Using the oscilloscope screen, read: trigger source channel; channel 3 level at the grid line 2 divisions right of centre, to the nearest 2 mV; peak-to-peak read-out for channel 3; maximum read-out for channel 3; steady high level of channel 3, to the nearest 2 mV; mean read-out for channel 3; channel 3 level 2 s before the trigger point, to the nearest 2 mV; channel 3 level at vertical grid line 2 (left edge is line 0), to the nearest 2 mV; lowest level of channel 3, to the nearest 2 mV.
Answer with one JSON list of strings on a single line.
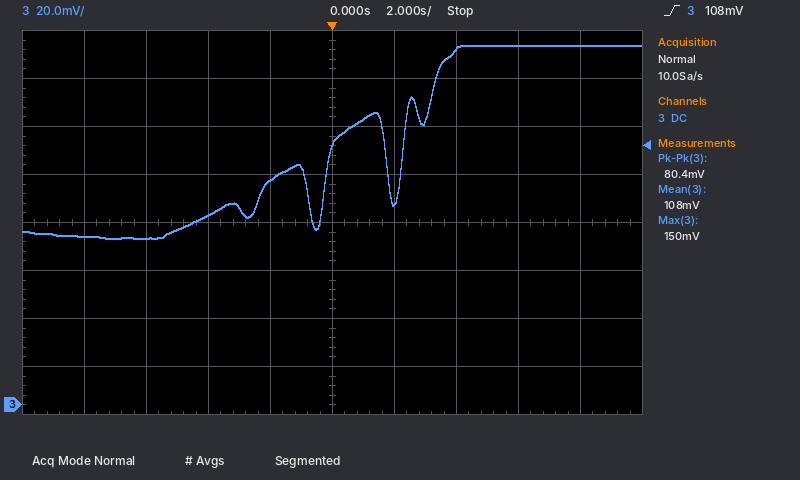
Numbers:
["channel 3", "148 mV", "80.4 mV", "150 mV", "150 mV", "108 mV", "94 mV", "70 mV", "70 mV"]
